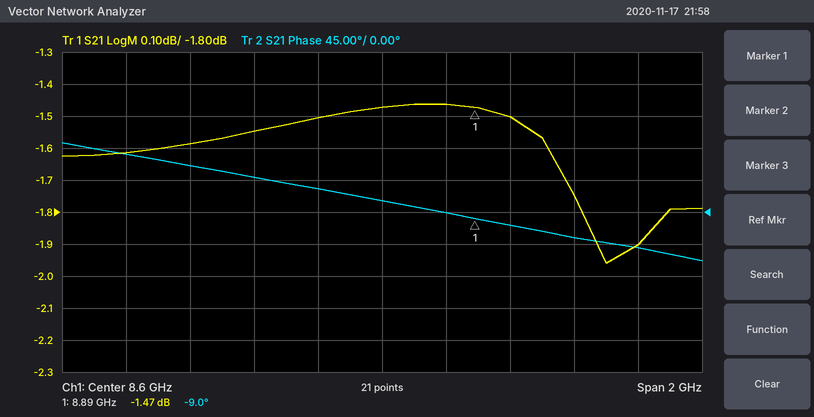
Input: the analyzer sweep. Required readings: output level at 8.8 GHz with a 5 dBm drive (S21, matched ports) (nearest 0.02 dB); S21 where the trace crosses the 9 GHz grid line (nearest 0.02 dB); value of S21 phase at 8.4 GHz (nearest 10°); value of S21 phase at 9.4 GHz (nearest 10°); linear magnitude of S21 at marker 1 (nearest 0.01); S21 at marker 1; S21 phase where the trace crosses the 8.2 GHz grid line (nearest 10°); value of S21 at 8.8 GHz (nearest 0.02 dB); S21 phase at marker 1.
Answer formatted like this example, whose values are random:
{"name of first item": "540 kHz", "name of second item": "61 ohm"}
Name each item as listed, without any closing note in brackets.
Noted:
{"output level at 8.8 GHz with a 5 dBm drive (S21, matched ports)": "3.54 dBm", "S21 where the trace crosses the 9 GHz grid line": "-1.50 dB", "value of S21 phase at 8.4 GHz": "30°", "value of S21 phase at 9.4 GHz": "-50°", "linear magnitude of S21 at marker 1": "0.84", "S21 at marker 1": "-1.47 dB", "S21 phase where the trace crosses the 8.2 GHz grid line": "50°", "value of S21 at 8.8 GHz": "-1.46 dB", "S21 phase at marker 1": "-9.0°"}
